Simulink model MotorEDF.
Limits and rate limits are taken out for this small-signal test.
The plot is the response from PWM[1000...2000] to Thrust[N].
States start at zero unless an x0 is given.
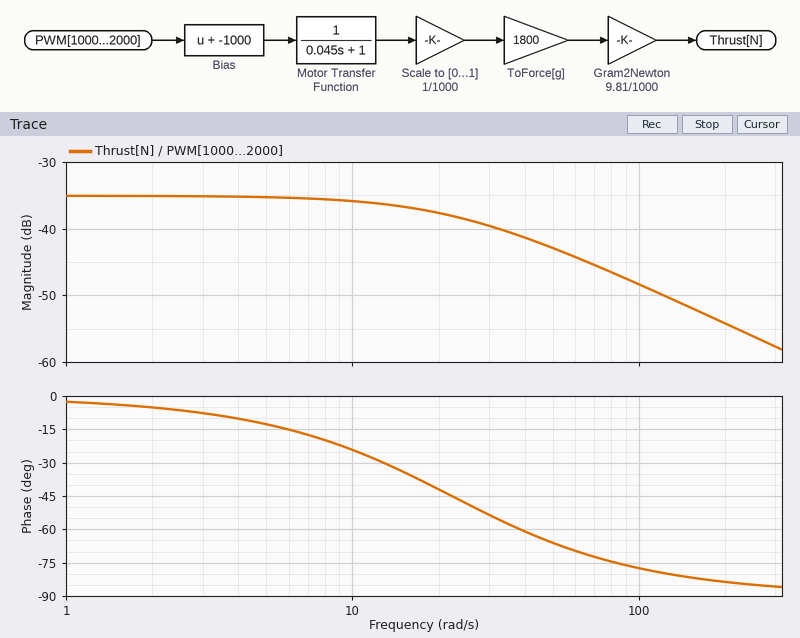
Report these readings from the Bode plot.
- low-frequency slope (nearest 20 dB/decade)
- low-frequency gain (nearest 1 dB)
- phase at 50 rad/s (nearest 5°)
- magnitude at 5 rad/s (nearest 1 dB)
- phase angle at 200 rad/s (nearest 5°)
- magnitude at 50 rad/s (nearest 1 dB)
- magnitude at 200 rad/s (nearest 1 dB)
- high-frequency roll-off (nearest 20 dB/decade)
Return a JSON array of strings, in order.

["0 dB/decade", "-35 dB", "-65°", "-35 dB", "-85°", "-43 dB", "-54 dB", "-20 dB/decade"]
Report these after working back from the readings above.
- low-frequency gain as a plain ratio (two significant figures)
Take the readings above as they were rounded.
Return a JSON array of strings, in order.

["0.018"]
